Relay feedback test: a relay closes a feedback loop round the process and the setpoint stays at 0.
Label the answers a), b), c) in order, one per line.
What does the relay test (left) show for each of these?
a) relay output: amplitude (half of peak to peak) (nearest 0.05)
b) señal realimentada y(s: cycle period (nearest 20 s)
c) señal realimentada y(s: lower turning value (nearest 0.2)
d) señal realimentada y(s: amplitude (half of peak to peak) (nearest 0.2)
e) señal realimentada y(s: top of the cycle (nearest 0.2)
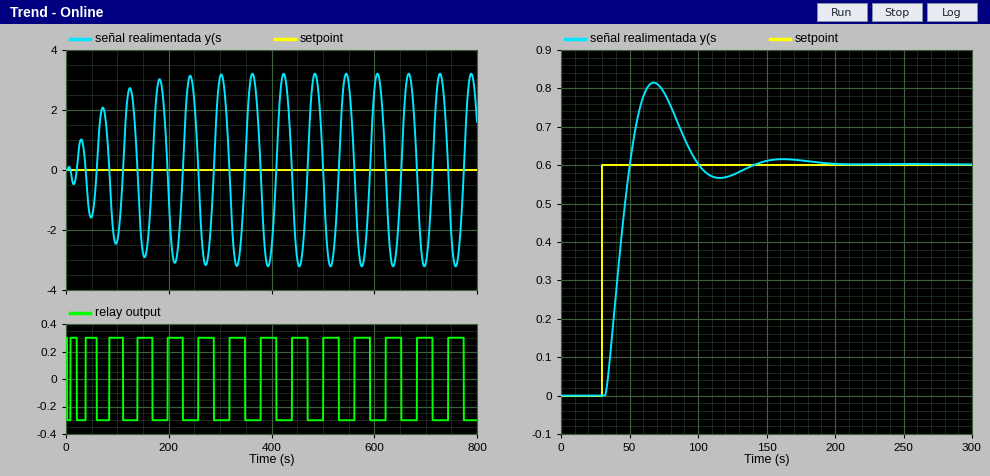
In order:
a) 0.30
b) 60 s
c) -3.2
d) 3.2
e) 3.2
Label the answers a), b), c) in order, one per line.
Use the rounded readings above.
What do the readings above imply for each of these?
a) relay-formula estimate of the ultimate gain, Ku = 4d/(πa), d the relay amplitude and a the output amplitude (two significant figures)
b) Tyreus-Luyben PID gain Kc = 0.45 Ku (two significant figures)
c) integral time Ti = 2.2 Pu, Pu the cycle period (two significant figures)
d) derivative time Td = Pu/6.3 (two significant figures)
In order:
a) 0.12
b) 0.054
c) 130 s
d) 9.5 s
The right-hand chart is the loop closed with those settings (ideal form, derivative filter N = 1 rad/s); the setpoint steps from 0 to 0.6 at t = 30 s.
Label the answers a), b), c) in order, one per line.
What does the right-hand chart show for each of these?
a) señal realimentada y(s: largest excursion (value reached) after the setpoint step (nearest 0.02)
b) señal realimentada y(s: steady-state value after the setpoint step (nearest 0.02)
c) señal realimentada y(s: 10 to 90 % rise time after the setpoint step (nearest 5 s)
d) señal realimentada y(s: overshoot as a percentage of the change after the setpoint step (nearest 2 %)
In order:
a) 0.82
b) 0.60
c) 15 s
d) 36 %
